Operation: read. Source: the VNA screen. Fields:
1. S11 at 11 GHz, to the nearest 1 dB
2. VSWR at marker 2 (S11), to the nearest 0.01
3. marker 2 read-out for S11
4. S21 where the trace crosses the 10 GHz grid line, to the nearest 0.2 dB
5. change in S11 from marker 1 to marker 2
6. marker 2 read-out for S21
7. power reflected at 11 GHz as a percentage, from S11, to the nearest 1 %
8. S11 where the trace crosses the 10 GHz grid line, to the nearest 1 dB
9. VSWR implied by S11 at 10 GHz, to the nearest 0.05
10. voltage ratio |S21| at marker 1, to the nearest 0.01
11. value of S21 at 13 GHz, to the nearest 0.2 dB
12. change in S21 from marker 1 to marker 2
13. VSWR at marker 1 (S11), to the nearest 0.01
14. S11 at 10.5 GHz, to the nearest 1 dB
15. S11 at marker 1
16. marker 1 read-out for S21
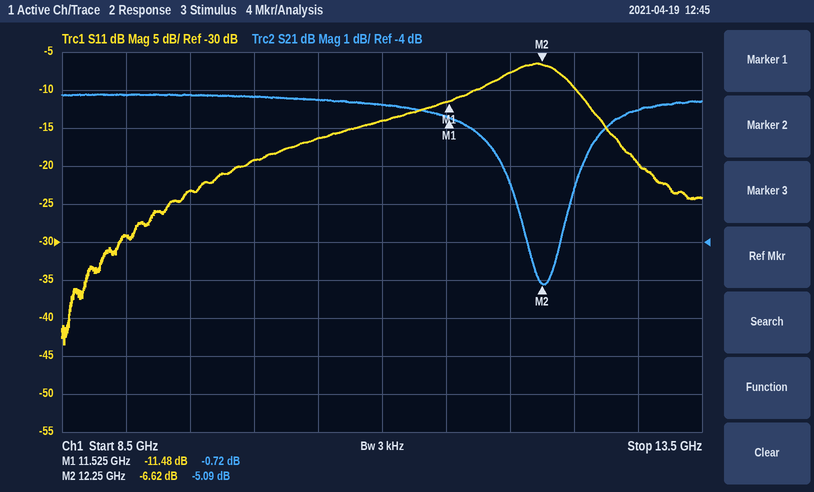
-14 dB
2.75
-6.62 dB
-0.2 dB
4.86 dB
-5.09 dB
4 %
-19 dB
1.25
0.92
-0.6 dB
-4.37 dB
1.73
-16 dB
-11.48 dB
-0.72 dB
